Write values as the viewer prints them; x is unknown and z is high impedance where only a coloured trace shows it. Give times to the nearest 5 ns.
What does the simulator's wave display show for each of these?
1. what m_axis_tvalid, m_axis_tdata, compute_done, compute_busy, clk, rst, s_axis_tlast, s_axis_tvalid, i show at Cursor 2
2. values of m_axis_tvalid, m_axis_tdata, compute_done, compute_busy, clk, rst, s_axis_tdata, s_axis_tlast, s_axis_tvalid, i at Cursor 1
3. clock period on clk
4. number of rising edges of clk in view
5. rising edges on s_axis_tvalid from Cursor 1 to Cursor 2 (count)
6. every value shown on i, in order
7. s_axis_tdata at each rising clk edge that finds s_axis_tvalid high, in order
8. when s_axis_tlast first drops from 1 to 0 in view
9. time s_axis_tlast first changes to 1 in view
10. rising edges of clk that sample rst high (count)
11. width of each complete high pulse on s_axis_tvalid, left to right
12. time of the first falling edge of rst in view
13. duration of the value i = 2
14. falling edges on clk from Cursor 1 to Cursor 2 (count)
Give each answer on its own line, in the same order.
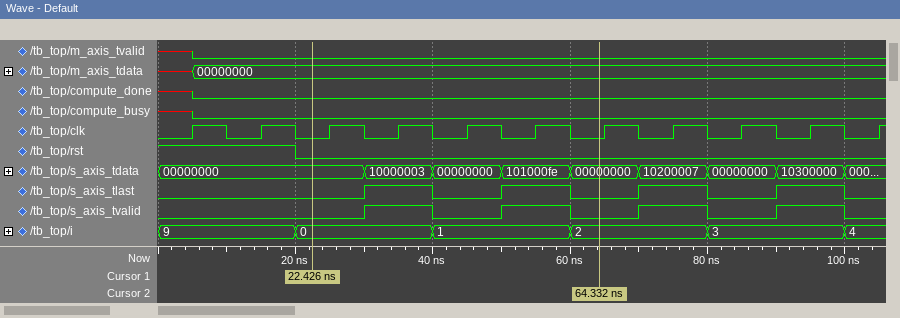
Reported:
m_axis_tvalid=0, m_axis_tdata=00000000, compute_done=0, compute_busy=0, clk=0, rst=0, s_axis_tlast=0, s_axis_tvalid=0, i=2
m_axis_tvalid=0, m_axis_tdata=00000000, compute_done=0, compute_busy=0, clk=0, rst=0, s_axis_tdata=00000000, s_axis_tlast=0, s_axis_tvalid=0, i=0
10 ns
11
2
9, 0, 1, 2, 3, 4
10000003, 101000fe, 10200007, 10300000
40 ns
30 ns
2
10 ns, 10 ns, 10 ns, 10 ns
20 ns
20 ns
4
